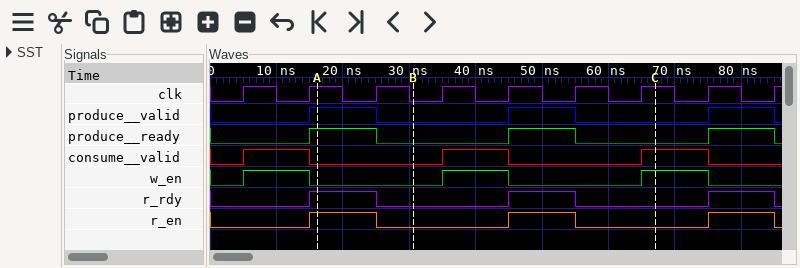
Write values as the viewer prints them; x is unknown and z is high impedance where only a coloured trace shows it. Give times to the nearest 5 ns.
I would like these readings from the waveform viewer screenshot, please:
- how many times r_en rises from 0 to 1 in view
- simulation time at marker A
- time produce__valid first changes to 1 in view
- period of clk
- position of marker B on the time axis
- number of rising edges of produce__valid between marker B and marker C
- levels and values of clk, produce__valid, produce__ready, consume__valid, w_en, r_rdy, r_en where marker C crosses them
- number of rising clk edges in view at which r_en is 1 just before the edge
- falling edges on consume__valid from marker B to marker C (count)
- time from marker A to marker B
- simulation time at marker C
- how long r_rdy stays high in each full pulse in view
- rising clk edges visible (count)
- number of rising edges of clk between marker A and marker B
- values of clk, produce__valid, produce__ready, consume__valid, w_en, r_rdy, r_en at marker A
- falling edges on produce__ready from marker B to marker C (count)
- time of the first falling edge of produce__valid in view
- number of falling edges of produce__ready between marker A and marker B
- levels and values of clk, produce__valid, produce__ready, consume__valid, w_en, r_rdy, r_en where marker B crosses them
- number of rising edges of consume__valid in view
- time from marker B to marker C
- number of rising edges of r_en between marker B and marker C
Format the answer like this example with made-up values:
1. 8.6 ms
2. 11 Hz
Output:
1. 3
2. 15 ns
3. 15 ns
4. 10 ns
5. 30 ns
6. 1
7. clk=1, produce__valid=0, produce__ready=0, consume__valid=1, w_en=1, r_rdy=0, r_en=0
8. 3
9. 1
10. 15 ns
11. 65 ns
12. 10 ns, 10 ns, 10 ns
13. 9
14. 1
15. clk=1, produce__valid=1, produce__ready=1, consume__valid=0, w_en=0, r_rdy=1, r_en=1
16. 1
17. 25 ns
18. 1
19. clk=0, produce__valid=0, produce__ready=0, consume__valid=0, w_en=0, r_rdy=0, r_en=0
20. 3
21. 35 ns
22. 1
